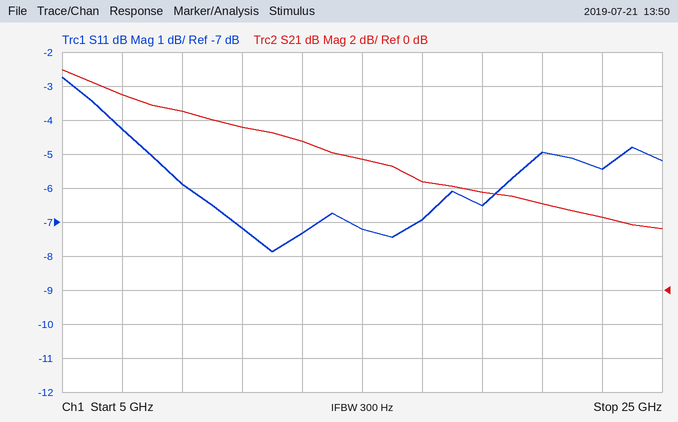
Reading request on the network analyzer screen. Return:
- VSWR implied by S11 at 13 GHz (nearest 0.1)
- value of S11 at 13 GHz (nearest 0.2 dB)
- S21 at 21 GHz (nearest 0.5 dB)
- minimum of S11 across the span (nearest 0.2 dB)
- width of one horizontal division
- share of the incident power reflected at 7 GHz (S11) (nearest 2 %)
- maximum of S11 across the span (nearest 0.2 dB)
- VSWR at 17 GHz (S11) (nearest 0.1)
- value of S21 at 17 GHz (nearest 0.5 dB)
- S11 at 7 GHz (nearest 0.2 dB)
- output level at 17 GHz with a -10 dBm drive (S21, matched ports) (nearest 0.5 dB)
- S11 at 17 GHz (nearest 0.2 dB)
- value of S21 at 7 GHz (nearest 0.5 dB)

2.5
-7.4 dB
5.0 dB
-7.8 dB
2 GHz
38 %
-2.8 dB
2.6
6.5 dB
-4.2 dB
-3.5 dBm
-7.0 dB
11.5 dB
